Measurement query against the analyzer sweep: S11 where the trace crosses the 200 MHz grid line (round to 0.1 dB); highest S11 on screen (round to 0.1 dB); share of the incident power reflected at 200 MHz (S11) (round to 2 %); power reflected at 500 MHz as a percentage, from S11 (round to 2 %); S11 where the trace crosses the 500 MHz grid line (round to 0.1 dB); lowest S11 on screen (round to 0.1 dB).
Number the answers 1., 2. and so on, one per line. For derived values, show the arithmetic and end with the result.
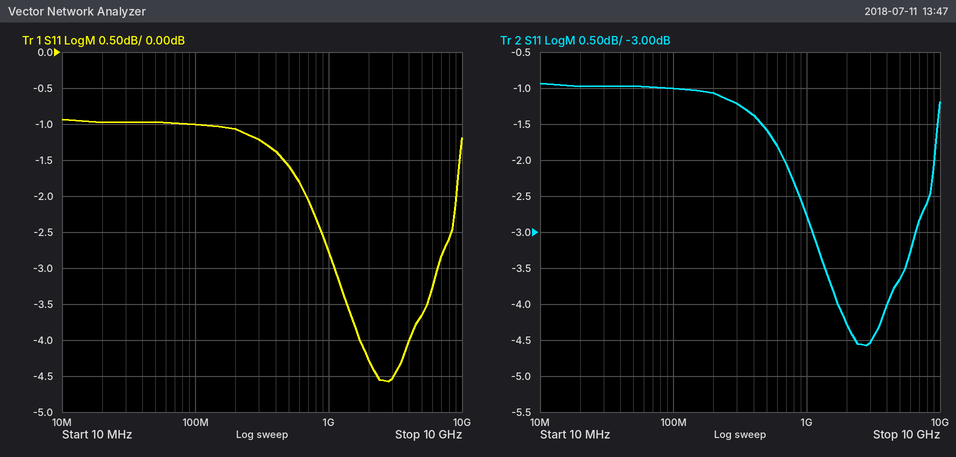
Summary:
1. -1.1 dB
2. -0.9 dB
3. 10^(-1.1/10) ≈ 78 %
4. 10^(-1.6/10) ≈ 69.2 %, so 70 % to the nearest 2 %
5. -1.6 dB
6. -4.6 dB
